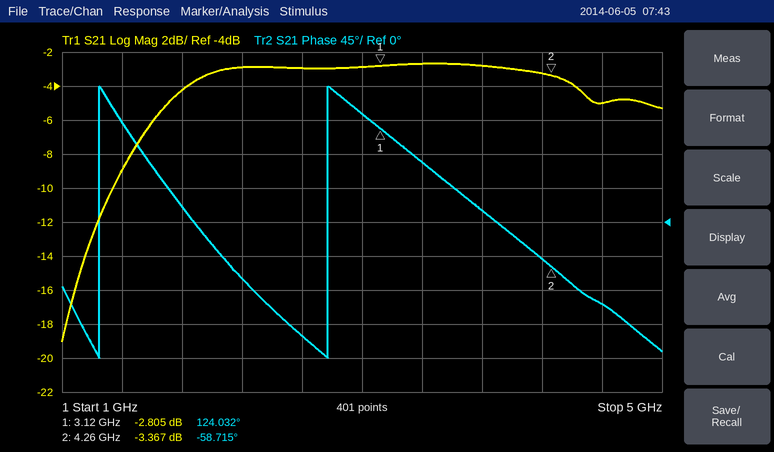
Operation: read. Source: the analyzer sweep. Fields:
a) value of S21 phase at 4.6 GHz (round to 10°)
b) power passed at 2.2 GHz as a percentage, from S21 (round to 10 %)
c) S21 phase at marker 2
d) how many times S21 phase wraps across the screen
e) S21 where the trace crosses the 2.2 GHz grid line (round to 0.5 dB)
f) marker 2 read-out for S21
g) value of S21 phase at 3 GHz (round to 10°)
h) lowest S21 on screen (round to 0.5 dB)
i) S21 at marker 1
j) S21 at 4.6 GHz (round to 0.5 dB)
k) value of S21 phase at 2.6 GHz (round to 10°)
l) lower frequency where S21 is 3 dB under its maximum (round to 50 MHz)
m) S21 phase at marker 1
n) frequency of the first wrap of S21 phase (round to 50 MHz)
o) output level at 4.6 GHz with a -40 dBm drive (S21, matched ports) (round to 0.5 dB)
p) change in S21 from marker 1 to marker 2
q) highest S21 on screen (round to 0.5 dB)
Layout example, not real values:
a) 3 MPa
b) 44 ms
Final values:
a) -110°
b) 50 %
c) -58.715°
d) 2
e) -3.0 dB
f) -3.367 dB
g) 140°
h) -19.0 dB
i) -2.805 dB
j) -5.0 dB
k) -150°
l) 1.65 GHz
m) 124.032°
n) 1.25 GHz
o) -45.0 dBm
p) -0.562 dB
q) -2.5 dB
